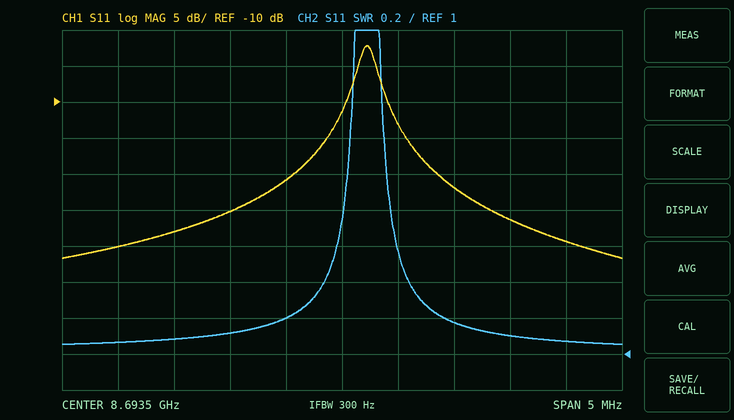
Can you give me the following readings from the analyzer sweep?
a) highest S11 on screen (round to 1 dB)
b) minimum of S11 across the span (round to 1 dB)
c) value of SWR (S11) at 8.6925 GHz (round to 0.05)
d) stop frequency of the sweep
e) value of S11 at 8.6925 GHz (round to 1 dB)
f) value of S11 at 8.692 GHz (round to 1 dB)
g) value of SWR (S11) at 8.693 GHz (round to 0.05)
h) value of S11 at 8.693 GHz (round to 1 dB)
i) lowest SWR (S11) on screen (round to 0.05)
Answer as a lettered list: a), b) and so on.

a) -2 dB
b) -32 dB
c) 1.10
d) 8.696 GHz
e) -25 dB
f) -28 dB
g) 1.20
h) -21 dB
i) 1.05
